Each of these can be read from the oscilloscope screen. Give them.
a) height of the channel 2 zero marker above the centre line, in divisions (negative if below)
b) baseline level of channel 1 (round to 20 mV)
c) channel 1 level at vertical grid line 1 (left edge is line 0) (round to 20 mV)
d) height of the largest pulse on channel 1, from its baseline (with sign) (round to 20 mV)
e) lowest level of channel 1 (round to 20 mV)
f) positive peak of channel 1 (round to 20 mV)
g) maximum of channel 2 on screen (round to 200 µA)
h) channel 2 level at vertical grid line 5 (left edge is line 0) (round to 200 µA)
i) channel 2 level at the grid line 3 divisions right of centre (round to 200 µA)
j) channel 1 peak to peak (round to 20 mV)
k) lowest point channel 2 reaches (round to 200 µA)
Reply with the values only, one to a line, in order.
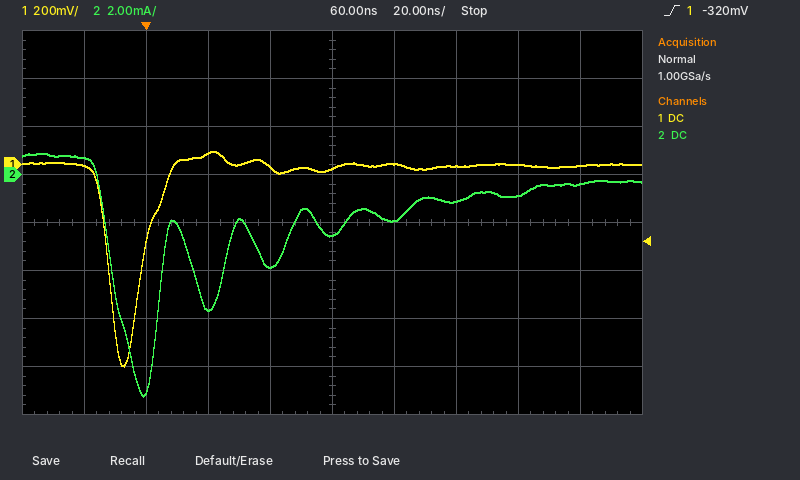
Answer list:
+1.0 div
0 mV
0 mV
-840 mV
-840 mV
60 mV
800 µA
-2.6 mA
-800 µA
900 mV
-9.2 mA
